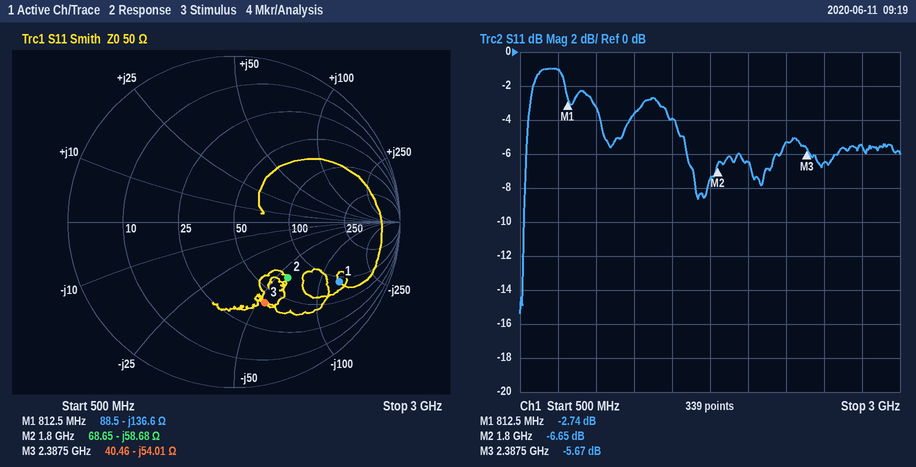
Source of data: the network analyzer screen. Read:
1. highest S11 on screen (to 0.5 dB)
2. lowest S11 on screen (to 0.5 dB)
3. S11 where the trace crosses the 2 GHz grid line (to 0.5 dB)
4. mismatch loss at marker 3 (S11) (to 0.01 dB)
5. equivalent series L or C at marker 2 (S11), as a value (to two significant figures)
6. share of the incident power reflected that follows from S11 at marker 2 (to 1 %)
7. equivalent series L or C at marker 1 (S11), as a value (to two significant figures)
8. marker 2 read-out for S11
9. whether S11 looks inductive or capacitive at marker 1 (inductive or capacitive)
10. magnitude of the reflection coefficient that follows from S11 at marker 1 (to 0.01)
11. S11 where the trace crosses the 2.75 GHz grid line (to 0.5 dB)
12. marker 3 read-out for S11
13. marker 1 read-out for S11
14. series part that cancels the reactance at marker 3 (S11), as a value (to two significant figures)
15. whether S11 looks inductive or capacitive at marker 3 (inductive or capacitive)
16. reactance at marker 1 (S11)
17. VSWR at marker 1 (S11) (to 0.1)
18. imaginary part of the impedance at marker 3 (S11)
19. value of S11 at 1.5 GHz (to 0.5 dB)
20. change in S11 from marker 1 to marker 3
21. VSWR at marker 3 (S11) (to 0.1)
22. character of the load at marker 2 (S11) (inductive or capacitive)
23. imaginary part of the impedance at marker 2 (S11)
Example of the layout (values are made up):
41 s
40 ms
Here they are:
-1.0 dB
-15.5 dB
-6.5 dB
1.37 dB
1.5 pF
22 %
1.4 pF
-6.65 dB
capacitive
0.73
-5.5 dB
-5.67 dB
-2.74 dB
3.6 nH
capacitive
-136.6 Ω
6.4
-54.01 Ω
-4.0 dB
-2.93 dB
3.2
capacitive
-58.68 Ω
